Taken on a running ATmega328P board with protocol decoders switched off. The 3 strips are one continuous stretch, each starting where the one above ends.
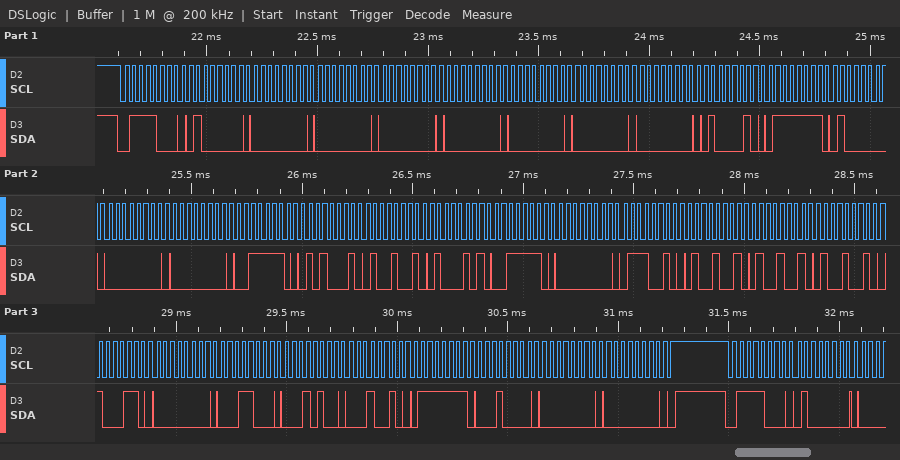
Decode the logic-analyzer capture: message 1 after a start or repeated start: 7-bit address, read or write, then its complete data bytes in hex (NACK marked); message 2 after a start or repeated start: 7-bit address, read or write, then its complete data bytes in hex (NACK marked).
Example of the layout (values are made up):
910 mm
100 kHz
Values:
0x3C write: 40 00 00 00 00 00 00 00 42 7F 40 00 00 3E 51 49 45 3E 00 72 49 49 49 46 00 18 14 12 7F 10 00 00
0x3C write: 40
